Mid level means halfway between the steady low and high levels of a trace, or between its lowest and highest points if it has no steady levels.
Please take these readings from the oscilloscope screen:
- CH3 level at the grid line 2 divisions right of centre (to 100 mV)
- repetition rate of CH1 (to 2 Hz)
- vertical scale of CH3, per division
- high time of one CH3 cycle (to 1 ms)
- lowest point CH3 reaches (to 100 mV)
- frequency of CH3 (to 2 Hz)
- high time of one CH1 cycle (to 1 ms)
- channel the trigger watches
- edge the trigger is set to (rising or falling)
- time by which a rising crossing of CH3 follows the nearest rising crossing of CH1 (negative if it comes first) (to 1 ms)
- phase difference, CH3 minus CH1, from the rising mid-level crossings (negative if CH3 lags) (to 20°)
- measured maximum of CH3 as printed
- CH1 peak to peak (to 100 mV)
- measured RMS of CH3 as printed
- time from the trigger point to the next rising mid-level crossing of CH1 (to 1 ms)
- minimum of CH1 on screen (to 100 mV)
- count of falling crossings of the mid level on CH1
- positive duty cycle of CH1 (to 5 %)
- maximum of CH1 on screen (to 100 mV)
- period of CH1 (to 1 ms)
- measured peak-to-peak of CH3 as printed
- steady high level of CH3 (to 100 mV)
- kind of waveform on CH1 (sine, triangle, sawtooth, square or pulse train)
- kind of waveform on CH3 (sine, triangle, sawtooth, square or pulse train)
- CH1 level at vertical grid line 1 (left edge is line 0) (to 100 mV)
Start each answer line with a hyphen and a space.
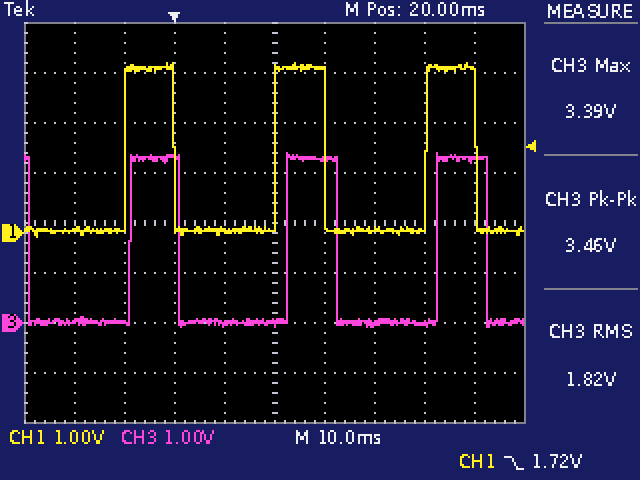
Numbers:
- 0.0 V
- 34 Hz
- 1 V
- 10 ms
- -100 mV
- 32 Hz
- 10 ms
- CH1
- falling
- +2 ms
- -20°
- 3.39 V
- 3.5 V
- 1.82 V
- 20 ms
- -100 mV
- 3
- 35 %
- 3.4 V
- 30 ms
- 3.46 V
- 3.3 V
- pulse train
- pulse train
- 100 mV
